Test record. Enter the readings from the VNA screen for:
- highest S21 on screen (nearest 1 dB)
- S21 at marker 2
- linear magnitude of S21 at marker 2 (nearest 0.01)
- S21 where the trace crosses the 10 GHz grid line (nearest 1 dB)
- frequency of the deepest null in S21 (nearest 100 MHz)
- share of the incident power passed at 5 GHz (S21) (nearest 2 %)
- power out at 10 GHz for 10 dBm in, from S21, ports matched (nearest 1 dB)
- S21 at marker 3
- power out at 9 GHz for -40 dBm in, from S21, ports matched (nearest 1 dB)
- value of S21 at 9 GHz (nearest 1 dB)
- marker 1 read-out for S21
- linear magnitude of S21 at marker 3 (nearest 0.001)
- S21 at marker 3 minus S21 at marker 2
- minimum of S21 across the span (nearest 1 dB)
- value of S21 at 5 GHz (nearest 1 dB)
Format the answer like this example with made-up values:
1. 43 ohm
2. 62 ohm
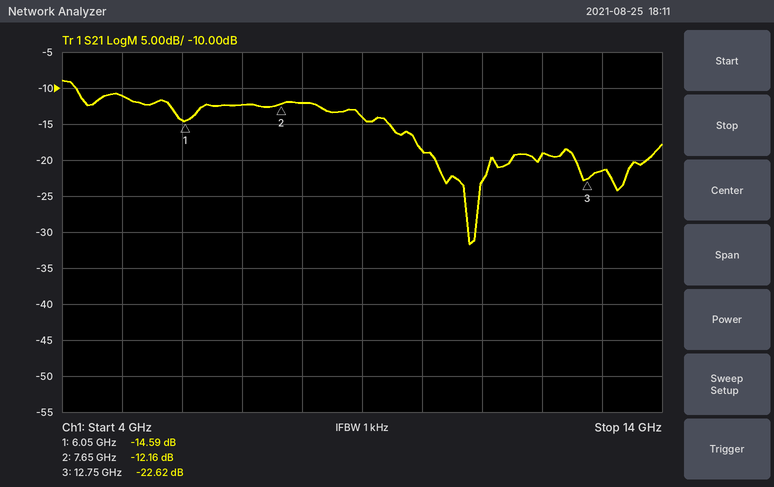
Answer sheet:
1. -9 dB
2. -12.16 dB
3. 0.25
4. -19 dB
5. 10.8 GHz
6. 8 %
7. -9 dBm
8. -22.62 dB
9. -54 dBm
10. -14 dB
11. -14.59 dB
12. 0.074
13. -10.46 dB
14. -32 dB
15. -11 dB
